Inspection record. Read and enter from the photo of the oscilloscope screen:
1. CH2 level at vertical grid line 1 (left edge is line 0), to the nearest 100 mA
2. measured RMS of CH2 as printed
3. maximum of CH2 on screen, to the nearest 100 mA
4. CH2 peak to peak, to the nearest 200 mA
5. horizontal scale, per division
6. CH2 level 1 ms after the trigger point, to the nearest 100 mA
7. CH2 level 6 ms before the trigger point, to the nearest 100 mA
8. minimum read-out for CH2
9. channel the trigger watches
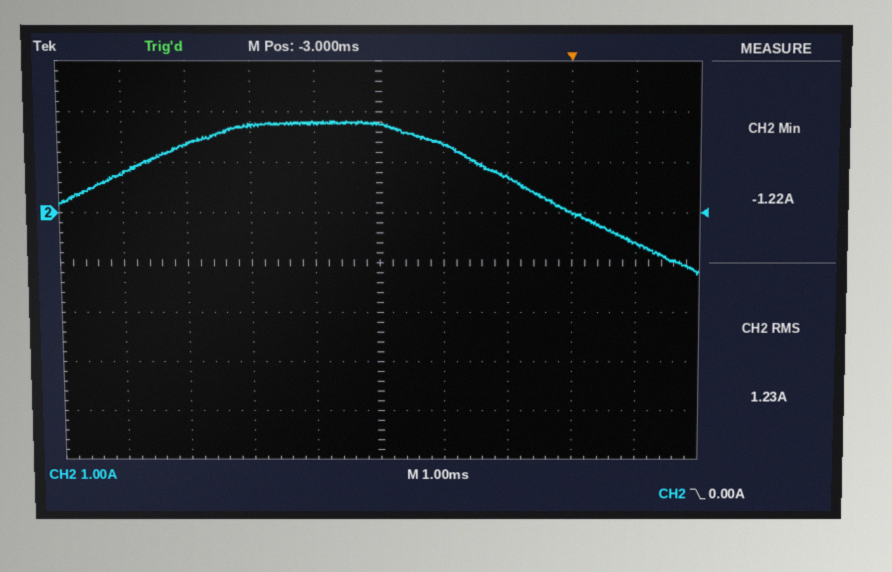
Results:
800 mA
1.23 A
1.8 A
3.0 A
1 ms
-600 mA
1.4 A
-1.22 A
CH2
